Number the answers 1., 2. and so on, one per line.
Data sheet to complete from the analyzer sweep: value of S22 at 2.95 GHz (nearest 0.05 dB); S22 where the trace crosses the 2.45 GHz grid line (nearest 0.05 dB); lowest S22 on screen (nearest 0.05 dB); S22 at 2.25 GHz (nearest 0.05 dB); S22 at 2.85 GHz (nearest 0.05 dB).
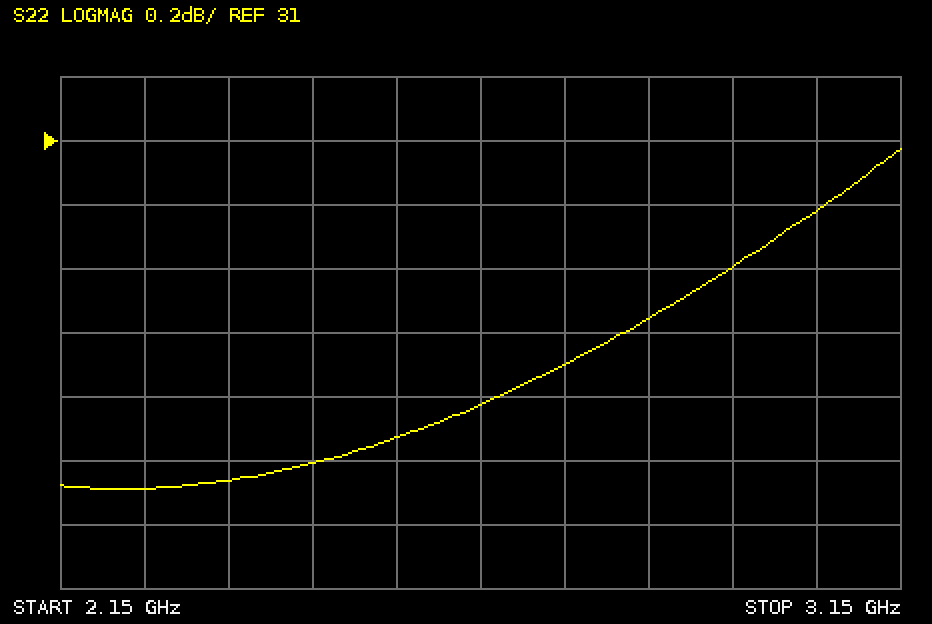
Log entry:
1. 30.60 dB
2. 30.00 dB
3. 29.90 dB
4. 29.90 dB
5. 30.45 dB
